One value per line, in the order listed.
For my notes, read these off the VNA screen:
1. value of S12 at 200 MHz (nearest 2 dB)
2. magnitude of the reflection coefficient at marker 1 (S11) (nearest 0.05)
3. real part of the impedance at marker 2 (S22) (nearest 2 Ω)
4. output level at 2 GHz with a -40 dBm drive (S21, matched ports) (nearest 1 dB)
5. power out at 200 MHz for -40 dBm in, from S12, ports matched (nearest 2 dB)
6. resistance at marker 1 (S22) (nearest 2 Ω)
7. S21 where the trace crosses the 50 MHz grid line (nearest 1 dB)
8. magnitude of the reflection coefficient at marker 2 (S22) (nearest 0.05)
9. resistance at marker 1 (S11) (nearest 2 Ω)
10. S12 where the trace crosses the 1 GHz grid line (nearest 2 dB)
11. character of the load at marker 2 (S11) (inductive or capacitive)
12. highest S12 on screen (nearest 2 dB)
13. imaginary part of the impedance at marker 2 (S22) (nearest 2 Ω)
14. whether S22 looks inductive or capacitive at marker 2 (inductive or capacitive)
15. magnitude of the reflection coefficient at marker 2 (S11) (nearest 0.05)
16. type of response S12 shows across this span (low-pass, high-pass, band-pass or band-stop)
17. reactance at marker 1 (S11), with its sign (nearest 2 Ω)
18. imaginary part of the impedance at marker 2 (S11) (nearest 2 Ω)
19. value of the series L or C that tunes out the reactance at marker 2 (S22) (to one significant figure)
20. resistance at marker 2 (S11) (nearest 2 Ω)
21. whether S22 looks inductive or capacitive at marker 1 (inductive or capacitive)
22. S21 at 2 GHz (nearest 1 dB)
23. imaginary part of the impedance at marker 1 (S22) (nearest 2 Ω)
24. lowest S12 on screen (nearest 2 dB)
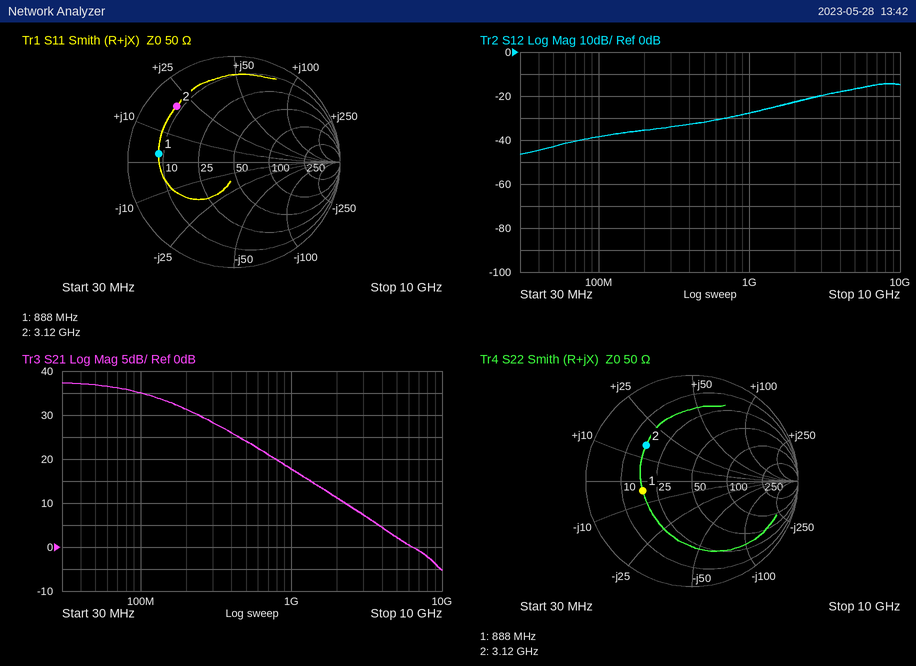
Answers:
-36 dB
0.70
16 Ω
-29 dBm
-76 dBm
18 Ω
37 dB
0.55
8 Ω
-28 dB
inductive
-14 dB
+16 Ω
inductive
0.75
high-pass
+2 Ω
+20 Ω
3 pF
8 Ω
capacitive
11 dB
-4 Ω
-46 dB
